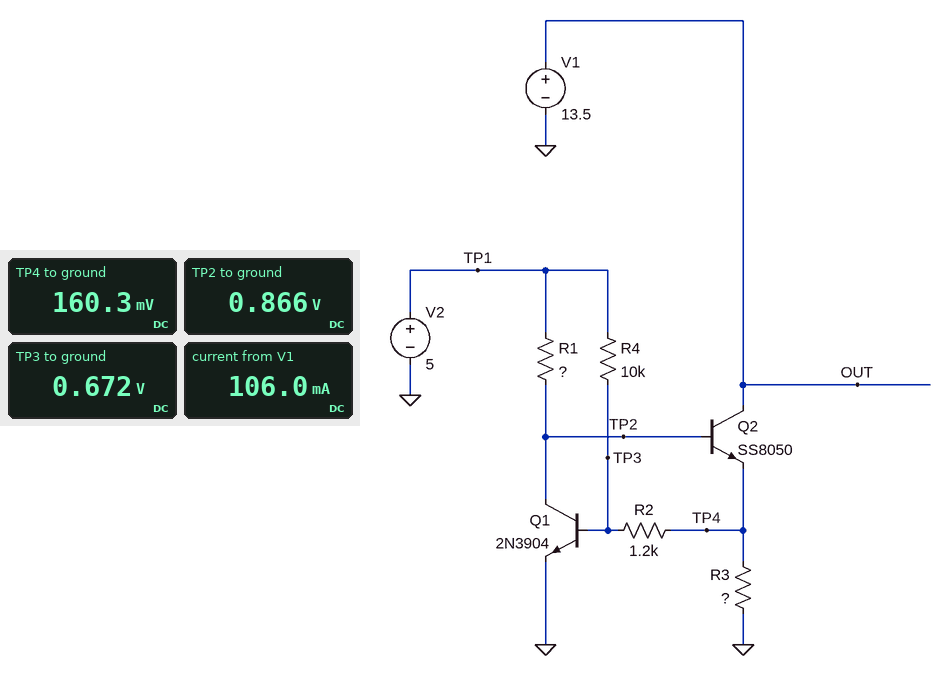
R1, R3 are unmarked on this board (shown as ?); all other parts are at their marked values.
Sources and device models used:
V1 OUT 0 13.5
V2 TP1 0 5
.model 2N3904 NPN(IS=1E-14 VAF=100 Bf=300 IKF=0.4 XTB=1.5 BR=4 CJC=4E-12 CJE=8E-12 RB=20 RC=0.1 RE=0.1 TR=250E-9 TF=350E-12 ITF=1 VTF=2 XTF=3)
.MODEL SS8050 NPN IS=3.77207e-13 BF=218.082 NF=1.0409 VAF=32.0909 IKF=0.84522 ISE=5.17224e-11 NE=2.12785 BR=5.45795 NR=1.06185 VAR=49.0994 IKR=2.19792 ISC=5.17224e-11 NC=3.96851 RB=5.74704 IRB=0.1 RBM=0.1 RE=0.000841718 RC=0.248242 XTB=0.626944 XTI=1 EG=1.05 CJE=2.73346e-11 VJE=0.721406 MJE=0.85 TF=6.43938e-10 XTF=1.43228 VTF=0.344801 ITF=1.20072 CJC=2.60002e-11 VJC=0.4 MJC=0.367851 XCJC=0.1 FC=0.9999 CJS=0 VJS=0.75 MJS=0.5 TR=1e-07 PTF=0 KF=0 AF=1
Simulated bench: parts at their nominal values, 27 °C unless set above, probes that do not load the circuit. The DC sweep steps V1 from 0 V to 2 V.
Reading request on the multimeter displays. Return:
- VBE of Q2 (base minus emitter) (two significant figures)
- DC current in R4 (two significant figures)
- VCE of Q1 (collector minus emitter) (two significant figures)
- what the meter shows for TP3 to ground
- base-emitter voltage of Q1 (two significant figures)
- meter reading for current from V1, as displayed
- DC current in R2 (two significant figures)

710 mV
430 µA
870 mV
0.672 V
670 mV
106.0 mA
430 µA
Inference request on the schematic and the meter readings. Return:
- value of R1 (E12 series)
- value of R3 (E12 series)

1.8 kΩ
1.5 Ω
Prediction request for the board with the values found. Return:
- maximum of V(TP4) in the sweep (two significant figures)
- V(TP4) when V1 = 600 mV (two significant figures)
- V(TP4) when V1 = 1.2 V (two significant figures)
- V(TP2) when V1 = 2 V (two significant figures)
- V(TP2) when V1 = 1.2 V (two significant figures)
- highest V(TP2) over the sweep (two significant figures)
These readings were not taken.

160 mV
160 mV
160 mV
870 mV
870 mV
870 mV
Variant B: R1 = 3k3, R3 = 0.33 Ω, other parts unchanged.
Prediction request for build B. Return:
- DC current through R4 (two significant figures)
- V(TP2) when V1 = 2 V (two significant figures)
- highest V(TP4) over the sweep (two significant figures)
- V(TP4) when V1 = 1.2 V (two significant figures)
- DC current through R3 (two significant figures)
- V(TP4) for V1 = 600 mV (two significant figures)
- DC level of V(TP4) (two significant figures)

440 µA
810 mV
68 mV
67 mV
260 mA
66 mV
86 mV
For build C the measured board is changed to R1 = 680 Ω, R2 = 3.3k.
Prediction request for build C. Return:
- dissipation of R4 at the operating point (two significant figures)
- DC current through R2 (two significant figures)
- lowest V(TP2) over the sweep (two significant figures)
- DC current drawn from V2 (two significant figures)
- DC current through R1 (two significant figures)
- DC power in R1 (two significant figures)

1.8 mW
220 µA
64 mV
7.7 mA
7.3 mA
36 mW
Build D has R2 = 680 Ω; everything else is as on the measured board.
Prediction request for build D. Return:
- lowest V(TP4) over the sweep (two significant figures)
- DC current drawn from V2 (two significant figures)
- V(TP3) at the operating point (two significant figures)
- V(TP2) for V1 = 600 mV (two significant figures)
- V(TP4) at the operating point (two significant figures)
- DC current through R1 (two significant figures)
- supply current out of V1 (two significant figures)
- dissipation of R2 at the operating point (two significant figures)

6.0 mV
2.6 mA
660 mV
1.1 V
370 mV
2.2 mA
240 mA
130 µW
